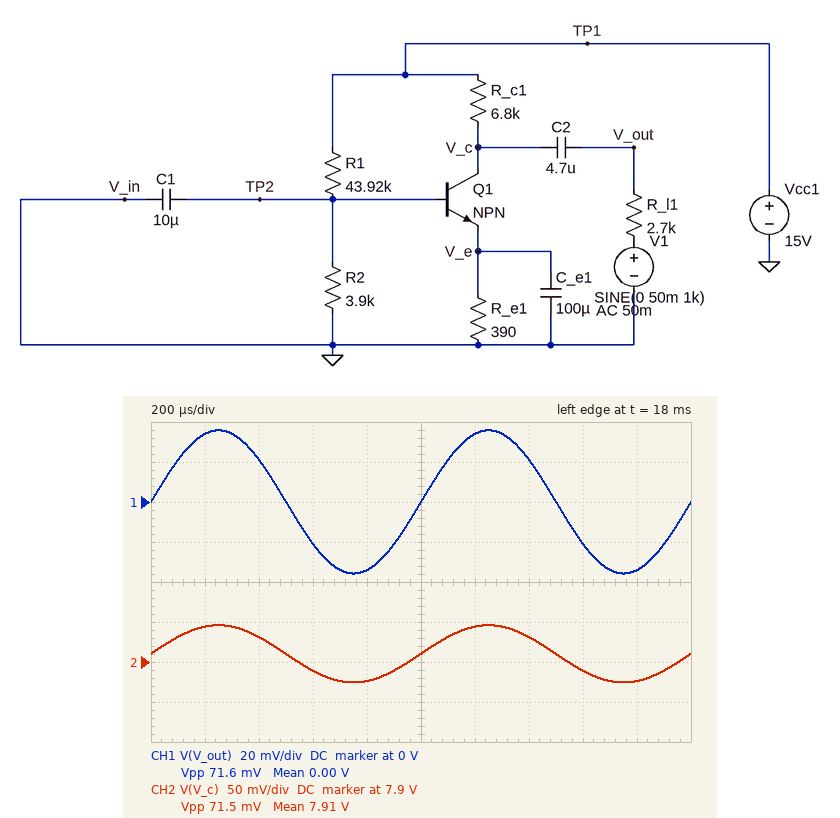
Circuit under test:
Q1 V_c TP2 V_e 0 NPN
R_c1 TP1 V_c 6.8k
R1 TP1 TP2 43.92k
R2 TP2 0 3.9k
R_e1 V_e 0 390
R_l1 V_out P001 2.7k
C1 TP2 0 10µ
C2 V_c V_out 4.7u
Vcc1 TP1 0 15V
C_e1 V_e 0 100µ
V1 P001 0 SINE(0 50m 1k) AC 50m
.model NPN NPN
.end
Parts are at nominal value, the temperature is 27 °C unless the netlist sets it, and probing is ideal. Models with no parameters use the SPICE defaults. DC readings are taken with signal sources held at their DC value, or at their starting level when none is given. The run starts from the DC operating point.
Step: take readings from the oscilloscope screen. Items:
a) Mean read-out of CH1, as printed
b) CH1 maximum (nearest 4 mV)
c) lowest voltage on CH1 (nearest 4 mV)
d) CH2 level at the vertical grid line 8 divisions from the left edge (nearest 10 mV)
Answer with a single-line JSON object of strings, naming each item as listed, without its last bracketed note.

{"Mean read-out of CH1, as printed": "0.00 V", "CH1 maximum": "36 mV", "lowest voltage on CH1": "-36 mV", "CH2 level at the vertical grid line 8 divisions from the left edge": "7.89 V"}
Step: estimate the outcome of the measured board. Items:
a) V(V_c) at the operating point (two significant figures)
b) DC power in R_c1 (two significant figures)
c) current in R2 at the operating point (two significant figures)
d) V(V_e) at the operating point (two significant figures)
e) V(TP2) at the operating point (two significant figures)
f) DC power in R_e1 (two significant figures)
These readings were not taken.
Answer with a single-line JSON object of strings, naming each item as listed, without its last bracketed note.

{"V(V_c) at the operating point": "7.9 V", "DC power in R_c1": "7.4 mW", "current in R2 at the operating point": "300 µA", "V(V_e) at the operating point": "410 mV", "V(TP2) at the operating point": "1.2 V", "DC power in R_e1": "430 µW"}
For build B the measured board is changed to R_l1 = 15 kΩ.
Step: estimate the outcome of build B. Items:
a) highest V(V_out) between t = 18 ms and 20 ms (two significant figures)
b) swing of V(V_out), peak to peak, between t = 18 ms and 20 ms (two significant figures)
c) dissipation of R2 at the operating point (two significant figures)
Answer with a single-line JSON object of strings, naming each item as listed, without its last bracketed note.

{"highest V(V_out) between t = 18 ms and 20 ms": "16 mV", "swing of V(V_out), peak to peak, between t = 18 ms and 20 ms": "31 mV", "dissipation of R2 at the operating point": "360 µW"}
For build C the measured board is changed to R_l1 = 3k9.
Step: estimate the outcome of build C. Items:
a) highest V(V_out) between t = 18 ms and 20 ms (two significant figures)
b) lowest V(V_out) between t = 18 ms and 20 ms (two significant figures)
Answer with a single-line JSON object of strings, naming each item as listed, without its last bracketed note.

{"highest V(V_out) between t = 18 ms and 20 ms": "32 mV", "lowest V(V_out) between t = 18 ms and 20 ms": "-32 mV"}
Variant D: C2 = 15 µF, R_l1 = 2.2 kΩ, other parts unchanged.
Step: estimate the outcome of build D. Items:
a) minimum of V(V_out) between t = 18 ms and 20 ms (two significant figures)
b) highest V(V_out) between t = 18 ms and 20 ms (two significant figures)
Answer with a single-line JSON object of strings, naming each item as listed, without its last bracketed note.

{"minimum of V(V_out) between t = 18 ms and 20 ms": "-38 mV", "highest V(V_out) between t = 18 ms and 20 ms": "38 mV"}
